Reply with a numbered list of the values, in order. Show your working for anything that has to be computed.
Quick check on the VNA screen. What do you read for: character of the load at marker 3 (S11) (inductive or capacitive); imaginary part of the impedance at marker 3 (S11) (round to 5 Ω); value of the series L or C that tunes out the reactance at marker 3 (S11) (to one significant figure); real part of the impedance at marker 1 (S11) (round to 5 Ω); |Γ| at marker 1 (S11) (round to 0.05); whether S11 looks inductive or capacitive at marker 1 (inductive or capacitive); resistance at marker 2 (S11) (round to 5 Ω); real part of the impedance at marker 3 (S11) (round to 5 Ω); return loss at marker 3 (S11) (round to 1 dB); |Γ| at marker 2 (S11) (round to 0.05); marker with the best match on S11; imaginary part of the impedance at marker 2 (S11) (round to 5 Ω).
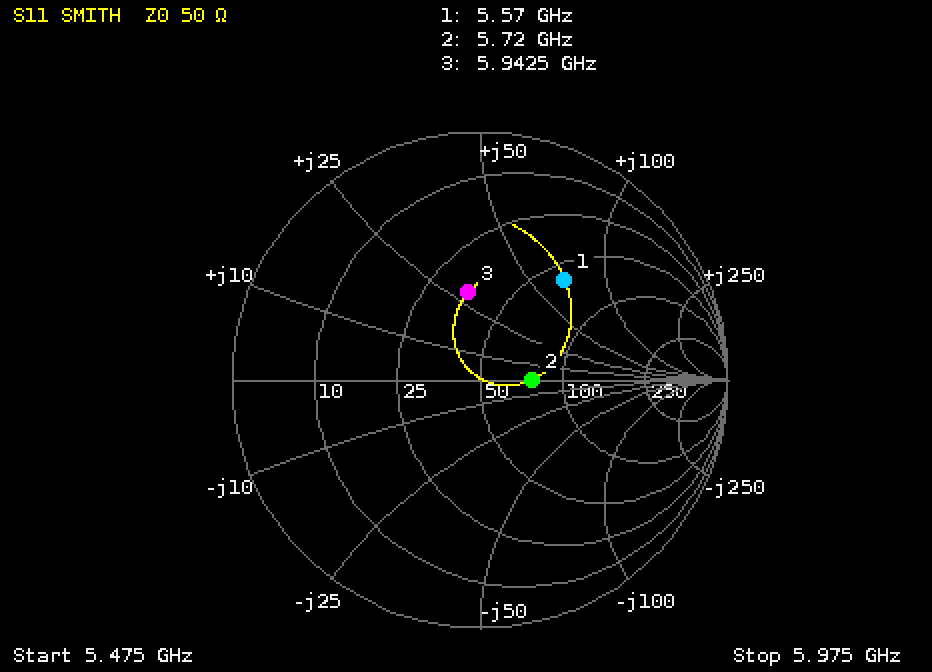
1. inductive
2. +30 Ω
3. C = 1/(2π × 5.9425 GHz × 30 Ω) ≈ 893 fF, so 900 fF to one significant figure
4. 60 Ω
5. 0.55
6. inductive
7. 75 Ω
8. 35 Ω
9. 9 dB
10. 0.20
11. marker 2
12. 0 Ω
